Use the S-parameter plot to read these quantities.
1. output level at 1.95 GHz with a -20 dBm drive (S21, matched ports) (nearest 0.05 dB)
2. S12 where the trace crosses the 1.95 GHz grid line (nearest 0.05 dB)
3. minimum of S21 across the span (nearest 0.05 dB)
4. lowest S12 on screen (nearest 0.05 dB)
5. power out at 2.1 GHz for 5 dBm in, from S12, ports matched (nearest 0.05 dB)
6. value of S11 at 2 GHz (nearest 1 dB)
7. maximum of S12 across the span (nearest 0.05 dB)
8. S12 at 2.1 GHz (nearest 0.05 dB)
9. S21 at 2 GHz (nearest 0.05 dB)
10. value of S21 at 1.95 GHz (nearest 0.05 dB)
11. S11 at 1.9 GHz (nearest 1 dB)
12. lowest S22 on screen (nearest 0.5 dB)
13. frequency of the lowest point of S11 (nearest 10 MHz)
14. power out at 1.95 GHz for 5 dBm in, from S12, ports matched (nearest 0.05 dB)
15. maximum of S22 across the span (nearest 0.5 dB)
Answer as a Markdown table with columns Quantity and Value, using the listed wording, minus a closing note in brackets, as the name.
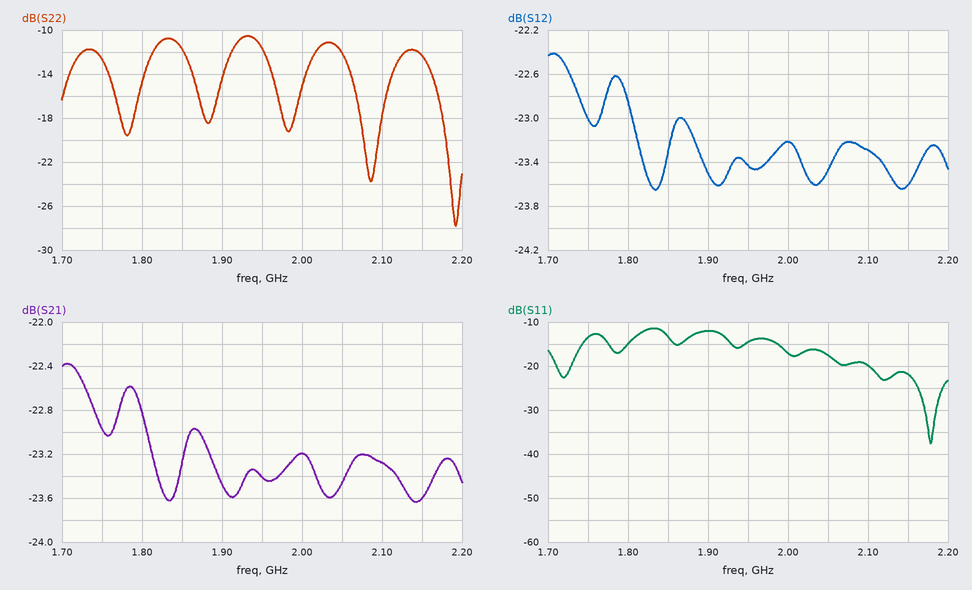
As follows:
| Quantity | Value |
|---|---|
| output level at 1.95 GHz with a -20 dBm drive (S21, matched ports) | -43.40 dBm |
| S12 where the trace crosses the 1.95 GHz grid line | -23.45 dB |
| minimum of S21 across the span | -23.65 dB |
| lowest S12 on screen | -23.65 dB |
| power out at 2.1 GHz for 5 dBm in, from S12, ports matched | -18.30 dBm |
| value of S11 at 2 GHz | -17 dB |
| maximum of S12 across the span | -22.40 dB |
| S12 at 2.1 GHz | -23.30 dB |
| S21 at 2 GHz | -23.20 dB |
| value of S21 at 1.95 GHz | -23.40 dB |
| S11 at 1.9 GHz | -12 dB |
| lowest S22 on screen | -28.0 dB |
| frequency of the lowest point of S11 | 2.18 GHz |
| power out at 1.95 GHz for 5 dBm in, from S12, ports matched | -18.45 dBm |
| maximum of S22 across the span | -10.5 dB |
